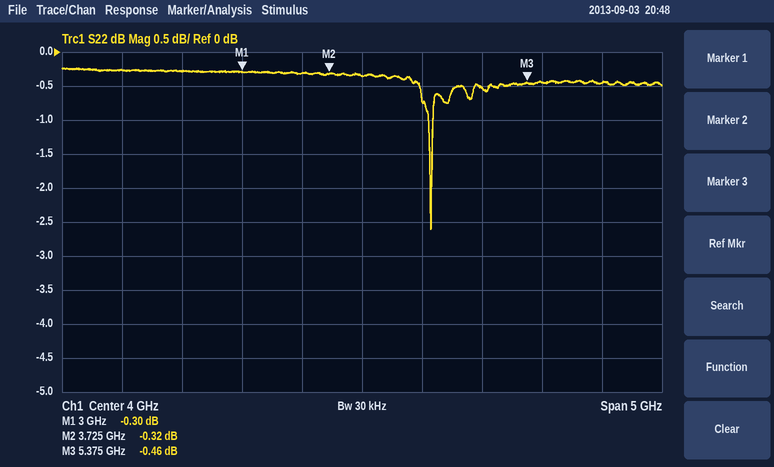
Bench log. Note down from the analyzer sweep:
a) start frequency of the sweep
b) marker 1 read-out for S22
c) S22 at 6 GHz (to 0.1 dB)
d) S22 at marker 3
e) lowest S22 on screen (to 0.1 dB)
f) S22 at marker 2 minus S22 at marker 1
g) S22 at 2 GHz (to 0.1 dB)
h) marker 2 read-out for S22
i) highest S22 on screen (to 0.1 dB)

1.5 GHz
-0.30 dB
-0.5 dB
-0.46 dB
-2.6 dB
-0.02 dB
-0.3 dB
-0.32 dB
-0.2 dB
